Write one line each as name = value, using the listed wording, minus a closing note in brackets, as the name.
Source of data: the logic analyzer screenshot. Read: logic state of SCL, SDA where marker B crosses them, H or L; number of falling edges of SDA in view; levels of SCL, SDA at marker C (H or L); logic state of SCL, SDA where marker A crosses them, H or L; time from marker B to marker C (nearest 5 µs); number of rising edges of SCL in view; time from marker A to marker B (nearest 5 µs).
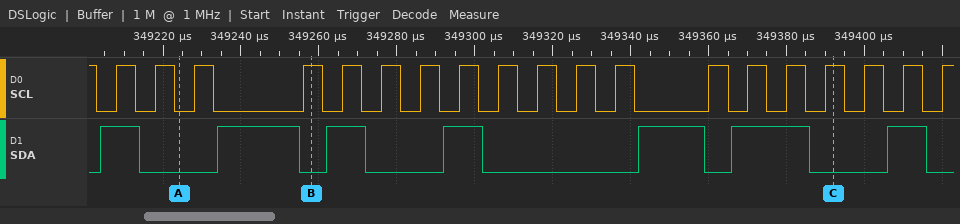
logic state of SCL, SDA where marker B crosses them, H or L = SCL=H, SDA=L
number of falling edges of SDA in view = 7
levels of SCL, SDA at marker C = SCL=H, SDA=L
logic state of SCL, SDA where marker A crosses them, H or L = SCL=L, SDA=L
time from marker B to marker C = 135 µs
number of rising edges of SCL in view = 19
time from marker A to marker B = 35 µs
